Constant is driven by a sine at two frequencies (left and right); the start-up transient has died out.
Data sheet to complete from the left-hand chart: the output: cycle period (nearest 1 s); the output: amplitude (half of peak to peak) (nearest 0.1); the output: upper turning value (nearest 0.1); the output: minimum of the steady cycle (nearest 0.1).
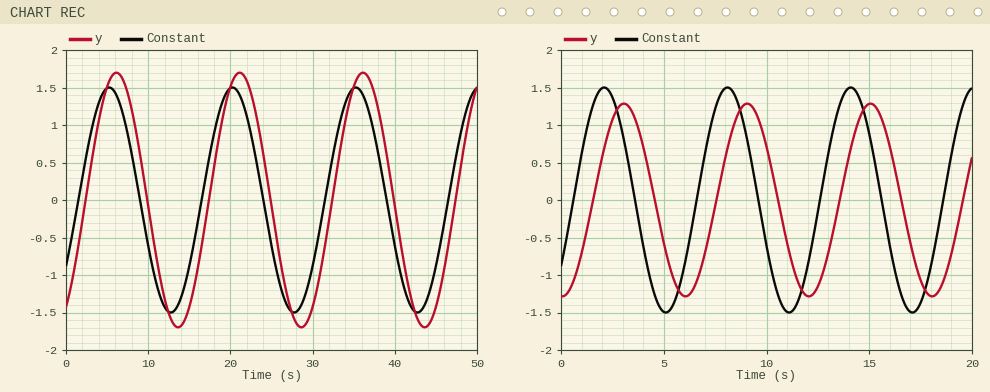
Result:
15 s
1.7
1.7
-1.7
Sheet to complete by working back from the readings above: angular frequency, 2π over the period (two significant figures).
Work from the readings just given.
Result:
0.42 rad/s
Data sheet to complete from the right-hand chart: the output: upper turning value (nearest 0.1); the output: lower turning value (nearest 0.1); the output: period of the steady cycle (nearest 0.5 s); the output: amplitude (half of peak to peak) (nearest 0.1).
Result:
1.3
-1.3
6.0 s
1.3
